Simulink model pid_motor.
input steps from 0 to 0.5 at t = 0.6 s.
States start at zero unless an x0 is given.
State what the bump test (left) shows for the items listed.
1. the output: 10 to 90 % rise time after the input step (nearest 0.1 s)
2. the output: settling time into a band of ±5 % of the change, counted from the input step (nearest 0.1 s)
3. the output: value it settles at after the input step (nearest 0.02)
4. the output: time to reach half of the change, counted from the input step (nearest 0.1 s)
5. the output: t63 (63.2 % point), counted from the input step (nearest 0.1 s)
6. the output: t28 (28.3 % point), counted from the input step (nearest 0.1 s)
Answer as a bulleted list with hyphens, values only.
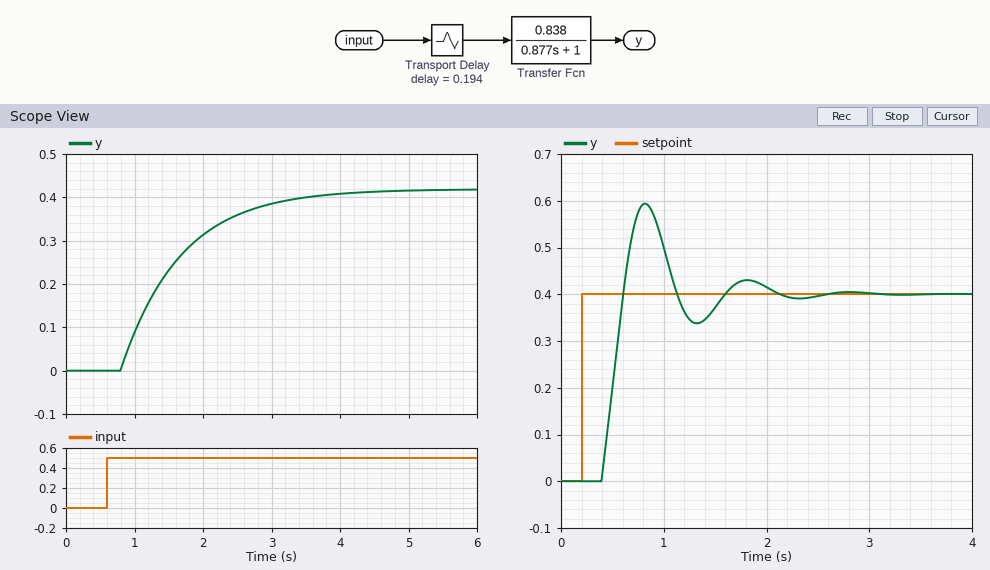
- 1.9 s
- 2.8 s
- 0.42
- 0.8 s
- 1.1 s
- 0.5 s
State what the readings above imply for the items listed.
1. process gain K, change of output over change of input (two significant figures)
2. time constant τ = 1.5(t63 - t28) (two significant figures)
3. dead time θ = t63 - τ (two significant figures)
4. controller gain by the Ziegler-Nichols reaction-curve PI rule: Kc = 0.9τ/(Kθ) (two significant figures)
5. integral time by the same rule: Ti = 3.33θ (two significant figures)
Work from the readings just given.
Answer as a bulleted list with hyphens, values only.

- 0.84
- 0.90 s
- 0.20 s
- 4.8
- 0.67 s
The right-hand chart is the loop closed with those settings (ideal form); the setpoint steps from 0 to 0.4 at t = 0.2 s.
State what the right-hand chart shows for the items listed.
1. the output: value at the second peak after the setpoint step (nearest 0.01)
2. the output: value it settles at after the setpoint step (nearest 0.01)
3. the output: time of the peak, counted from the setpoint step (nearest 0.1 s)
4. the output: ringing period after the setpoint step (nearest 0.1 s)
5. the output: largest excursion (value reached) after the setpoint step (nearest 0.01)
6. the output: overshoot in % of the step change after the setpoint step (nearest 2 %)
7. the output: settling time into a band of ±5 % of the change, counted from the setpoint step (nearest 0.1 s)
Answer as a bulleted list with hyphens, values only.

- 0.43
- 0.40
- 0.6 s
- 1.0 s
- 0.59
- 48 %
- 1.8 s
